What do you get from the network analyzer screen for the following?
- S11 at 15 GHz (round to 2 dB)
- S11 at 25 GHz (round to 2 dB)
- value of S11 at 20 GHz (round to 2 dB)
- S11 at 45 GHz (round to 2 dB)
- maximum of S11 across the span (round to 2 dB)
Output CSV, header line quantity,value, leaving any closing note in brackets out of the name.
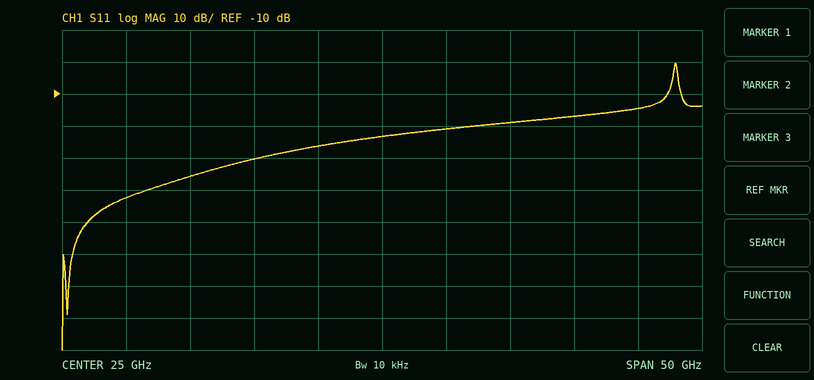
quantity,value
S11 at 15 GHz,-30 dB
S11 at 25 GHz,-24 dB
value of S11 at 20 GHz,-26 dB
S11 at 45 GHz,-14 dB
maximum of S11 across the span,0 dB
